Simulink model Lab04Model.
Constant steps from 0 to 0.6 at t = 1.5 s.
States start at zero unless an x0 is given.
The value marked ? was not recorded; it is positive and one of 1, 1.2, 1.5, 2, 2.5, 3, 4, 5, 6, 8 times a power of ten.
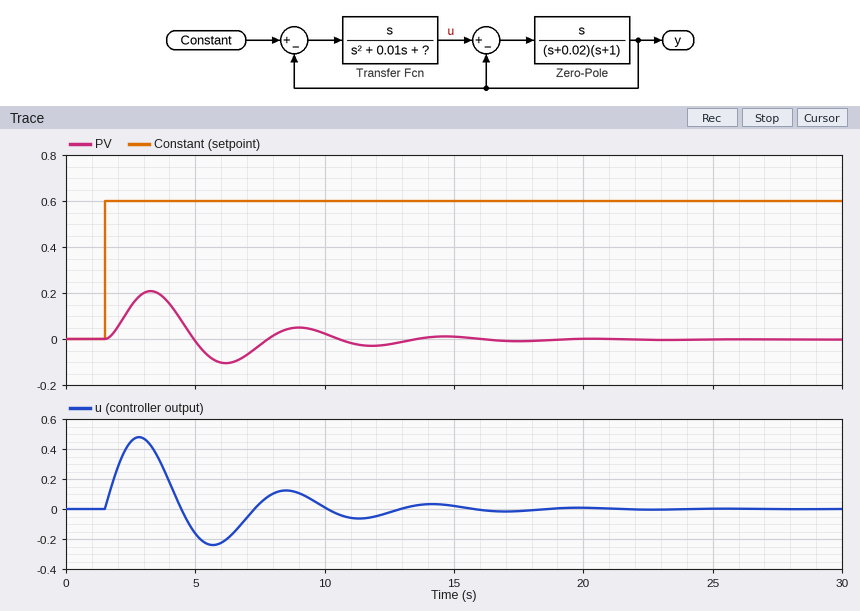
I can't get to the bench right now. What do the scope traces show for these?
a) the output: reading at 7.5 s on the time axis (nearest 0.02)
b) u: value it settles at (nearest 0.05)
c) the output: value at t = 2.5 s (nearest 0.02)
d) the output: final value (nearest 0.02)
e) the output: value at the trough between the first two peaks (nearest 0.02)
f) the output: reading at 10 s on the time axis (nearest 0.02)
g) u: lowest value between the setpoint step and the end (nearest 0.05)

-0.02
0.00
0.14
0.00
-0.10
0.02
-0.25
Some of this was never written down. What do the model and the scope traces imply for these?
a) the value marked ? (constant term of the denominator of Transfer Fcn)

1
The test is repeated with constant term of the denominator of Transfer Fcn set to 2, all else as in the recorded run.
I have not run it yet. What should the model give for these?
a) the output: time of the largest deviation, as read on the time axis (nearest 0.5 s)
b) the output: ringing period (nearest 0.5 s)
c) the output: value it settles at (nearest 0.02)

3.0 s
4.0 s
0.00
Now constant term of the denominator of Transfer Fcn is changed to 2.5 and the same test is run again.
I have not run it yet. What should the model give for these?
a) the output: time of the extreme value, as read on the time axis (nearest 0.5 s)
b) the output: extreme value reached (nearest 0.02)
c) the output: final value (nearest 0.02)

3.0 s
0.14
0.00
